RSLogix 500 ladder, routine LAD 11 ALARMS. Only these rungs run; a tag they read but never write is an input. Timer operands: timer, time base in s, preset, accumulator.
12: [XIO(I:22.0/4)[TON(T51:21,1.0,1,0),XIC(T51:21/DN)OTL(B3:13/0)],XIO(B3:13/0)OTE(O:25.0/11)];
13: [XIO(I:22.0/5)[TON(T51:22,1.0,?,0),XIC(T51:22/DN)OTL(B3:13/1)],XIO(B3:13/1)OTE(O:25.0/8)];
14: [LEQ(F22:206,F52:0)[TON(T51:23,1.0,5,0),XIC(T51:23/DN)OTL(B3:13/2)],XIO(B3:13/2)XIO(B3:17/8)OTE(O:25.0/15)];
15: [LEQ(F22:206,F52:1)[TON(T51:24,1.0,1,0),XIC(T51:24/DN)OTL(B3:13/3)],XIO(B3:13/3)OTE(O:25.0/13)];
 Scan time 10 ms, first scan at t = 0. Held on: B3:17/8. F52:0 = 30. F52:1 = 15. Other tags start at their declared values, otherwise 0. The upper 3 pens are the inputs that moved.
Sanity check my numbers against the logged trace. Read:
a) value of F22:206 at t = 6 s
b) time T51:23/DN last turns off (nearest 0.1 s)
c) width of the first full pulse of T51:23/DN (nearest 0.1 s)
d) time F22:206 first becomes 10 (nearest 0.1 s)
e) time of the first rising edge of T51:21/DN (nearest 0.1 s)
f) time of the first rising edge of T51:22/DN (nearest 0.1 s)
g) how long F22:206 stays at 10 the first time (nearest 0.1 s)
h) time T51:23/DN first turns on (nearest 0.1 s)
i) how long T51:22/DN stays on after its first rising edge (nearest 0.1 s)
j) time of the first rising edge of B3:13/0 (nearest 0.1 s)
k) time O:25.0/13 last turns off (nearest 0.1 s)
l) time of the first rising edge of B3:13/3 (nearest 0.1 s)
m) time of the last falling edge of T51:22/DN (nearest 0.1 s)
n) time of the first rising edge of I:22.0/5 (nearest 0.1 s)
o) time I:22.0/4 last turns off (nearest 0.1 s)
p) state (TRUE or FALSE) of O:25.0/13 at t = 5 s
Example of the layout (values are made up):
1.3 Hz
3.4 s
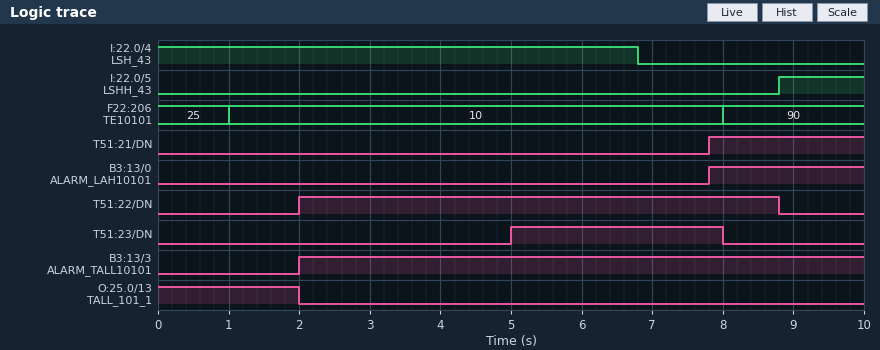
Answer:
10
8.0 s
3.0 s
1.0 s
7.8 s
2.0 s
7.0 s
5.0 s
6.8 s
7.8 s
2.0 s
2.0 s
8.8 s
8.8 s
6.8 s
FALSE
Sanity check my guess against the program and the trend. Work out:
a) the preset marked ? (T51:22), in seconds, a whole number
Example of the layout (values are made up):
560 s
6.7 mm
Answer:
2 s
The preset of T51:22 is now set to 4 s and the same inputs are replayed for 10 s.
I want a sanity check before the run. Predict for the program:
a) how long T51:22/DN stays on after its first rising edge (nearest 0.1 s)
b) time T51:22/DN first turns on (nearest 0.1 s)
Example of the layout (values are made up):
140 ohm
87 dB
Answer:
4.8 s
4.0 s
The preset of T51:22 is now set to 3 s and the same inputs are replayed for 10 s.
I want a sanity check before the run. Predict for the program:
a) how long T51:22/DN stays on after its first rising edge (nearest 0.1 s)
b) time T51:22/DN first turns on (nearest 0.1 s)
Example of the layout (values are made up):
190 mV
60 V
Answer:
5.8 s
3.0 s
